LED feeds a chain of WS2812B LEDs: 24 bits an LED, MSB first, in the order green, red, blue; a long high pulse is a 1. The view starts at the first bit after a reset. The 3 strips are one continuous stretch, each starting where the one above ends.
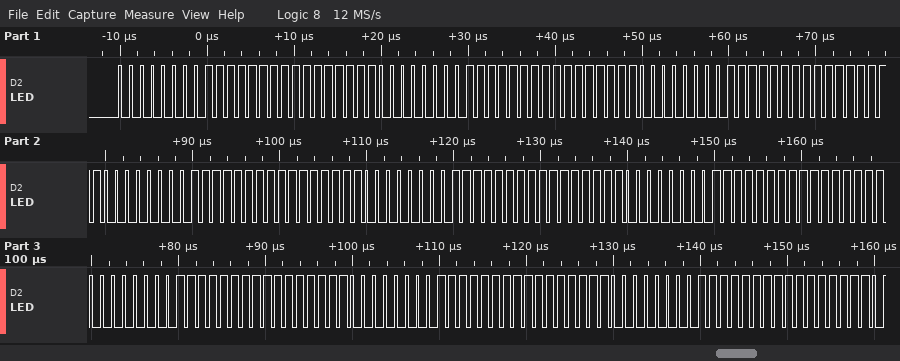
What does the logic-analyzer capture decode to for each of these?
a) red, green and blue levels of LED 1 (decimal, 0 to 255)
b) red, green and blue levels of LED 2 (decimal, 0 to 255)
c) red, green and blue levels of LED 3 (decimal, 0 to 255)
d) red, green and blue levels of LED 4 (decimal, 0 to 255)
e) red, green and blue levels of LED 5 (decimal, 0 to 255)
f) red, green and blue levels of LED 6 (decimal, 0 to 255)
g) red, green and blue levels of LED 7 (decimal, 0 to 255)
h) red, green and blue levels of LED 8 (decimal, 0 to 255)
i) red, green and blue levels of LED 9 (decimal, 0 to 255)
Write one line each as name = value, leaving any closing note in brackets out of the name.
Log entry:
red, green and blue levels of LED 1 = 255, 0, 255
red, green and blue levels of LED 2 = 255, 0, 255
red, green and blue levels of LED 3 = 255, 0, 255
red, green and blue levels of LED 4 = 255, 0, 255
red, green and blue levels of LED 5 = 255, 0, 255
red, green and blue levels of LED 6 = 255, 0, 255
red, green and blue levels of LED 7 = 255, 0, 255
red, green and blue levels of LED 8 = 255, 0, 255
red, green and blue levels of LED 9 = 255, 0, 255
